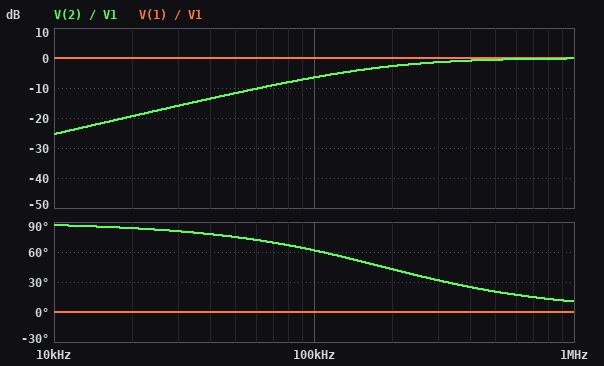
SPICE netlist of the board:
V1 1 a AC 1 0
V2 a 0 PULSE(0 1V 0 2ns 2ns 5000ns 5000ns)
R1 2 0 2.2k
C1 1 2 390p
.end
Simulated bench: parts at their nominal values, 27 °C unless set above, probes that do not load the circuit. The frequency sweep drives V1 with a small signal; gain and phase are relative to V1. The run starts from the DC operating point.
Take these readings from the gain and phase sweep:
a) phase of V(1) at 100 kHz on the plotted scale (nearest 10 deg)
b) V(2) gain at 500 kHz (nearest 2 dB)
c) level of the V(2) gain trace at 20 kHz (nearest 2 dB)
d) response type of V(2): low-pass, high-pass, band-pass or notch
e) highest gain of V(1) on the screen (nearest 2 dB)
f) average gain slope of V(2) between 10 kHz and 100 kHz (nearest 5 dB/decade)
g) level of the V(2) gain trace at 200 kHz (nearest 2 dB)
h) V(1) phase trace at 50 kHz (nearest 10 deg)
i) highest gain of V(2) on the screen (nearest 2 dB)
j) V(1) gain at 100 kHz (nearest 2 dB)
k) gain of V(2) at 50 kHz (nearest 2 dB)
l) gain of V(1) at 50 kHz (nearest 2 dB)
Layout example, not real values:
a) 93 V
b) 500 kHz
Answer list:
a) 0 deg
b) 0 dB
c) -20 dB
d) high-pass
e) 0 dB
f) 20 dB/decade
g) -2 dB
h) 0 deg
i) 0 dB
j) 0 dB
k) -12 dB
l) 0 dB
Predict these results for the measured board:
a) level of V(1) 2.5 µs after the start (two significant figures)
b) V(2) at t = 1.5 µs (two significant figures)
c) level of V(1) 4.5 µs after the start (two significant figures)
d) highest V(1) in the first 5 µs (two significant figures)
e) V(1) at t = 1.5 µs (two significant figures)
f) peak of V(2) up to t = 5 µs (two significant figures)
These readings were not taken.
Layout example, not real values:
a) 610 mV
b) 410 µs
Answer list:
a) 1.0 V
b) 170 mV
c) 1.0 V
d) 1.0 V
e) 1.0 V
f) 1.0 V
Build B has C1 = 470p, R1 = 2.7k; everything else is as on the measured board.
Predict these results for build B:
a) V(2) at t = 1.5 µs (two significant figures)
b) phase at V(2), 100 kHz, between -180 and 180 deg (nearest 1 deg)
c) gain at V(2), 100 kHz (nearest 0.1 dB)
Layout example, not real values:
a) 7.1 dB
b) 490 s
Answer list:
a) 310 mV
b) 51 deg
c) -4.1 dB
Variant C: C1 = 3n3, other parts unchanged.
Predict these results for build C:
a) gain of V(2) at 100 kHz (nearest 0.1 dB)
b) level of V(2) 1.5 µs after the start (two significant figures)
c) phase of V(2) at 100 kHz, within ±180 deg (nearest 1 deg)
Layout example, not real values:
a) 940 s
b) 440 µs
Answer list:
a) -0.2 dB
b) 810 mV
c) 12 deg
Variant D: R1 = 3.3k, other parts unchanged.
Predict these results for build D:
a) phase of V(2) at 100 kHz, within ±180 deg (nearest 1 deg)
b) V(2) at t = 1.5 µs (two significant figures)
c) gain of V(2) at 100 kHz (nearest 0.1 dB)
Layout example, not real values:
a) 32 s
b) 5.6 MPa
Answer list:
a) 51 deg
b) 310 mV
c) -4.0 dB
